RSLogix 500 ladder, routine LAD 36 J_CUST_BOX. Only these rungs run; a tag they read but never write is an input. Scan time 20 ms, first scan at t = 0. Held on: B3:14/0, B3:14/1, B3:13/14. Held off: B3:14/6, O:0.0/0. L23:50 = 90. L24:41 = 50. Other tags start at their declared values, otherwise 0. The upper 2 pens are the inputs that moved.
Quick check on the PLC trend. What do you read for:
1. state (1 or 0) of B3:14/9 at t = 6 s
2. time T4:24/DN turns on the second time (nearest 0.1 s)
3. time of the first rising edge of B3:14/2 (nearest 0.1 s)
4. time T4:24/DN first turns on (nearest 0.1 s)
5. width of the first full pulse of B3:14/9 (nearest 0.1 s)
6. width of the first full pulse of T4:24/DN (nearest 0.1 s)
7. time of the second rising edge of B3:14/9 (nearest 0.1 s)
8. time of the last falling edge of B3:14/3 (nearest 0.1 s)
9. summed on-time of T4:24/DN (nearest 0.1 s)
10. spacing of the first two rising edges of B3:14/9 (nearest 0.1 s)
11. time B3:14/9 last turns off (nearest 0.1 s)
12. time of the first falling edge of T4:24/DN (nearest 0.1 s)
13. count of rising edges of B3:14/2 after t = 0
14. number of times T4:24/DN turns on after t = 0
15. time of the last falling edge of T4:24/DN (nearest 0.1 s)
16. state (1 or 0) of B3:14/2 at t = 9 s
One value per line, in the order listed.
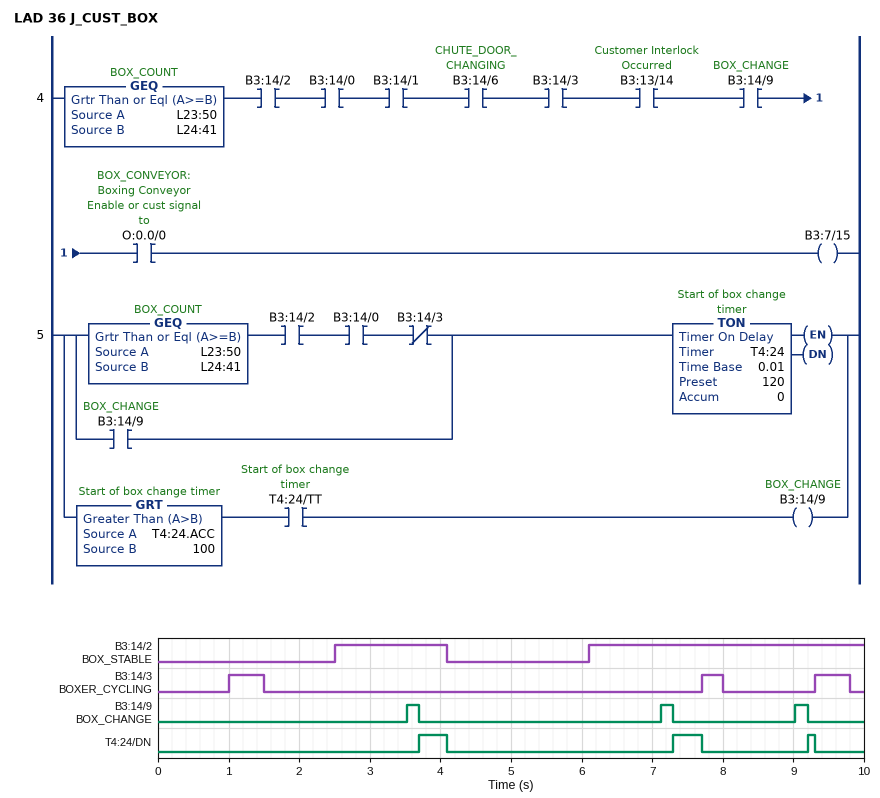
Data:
0
7.3 s
2.5 s
3.7 s
0.2 s
0.4 s
7.1 s
9.8 s
0.9 s
3.6 s
9.2 s
4.1 s
2
3
9.3 s
1
